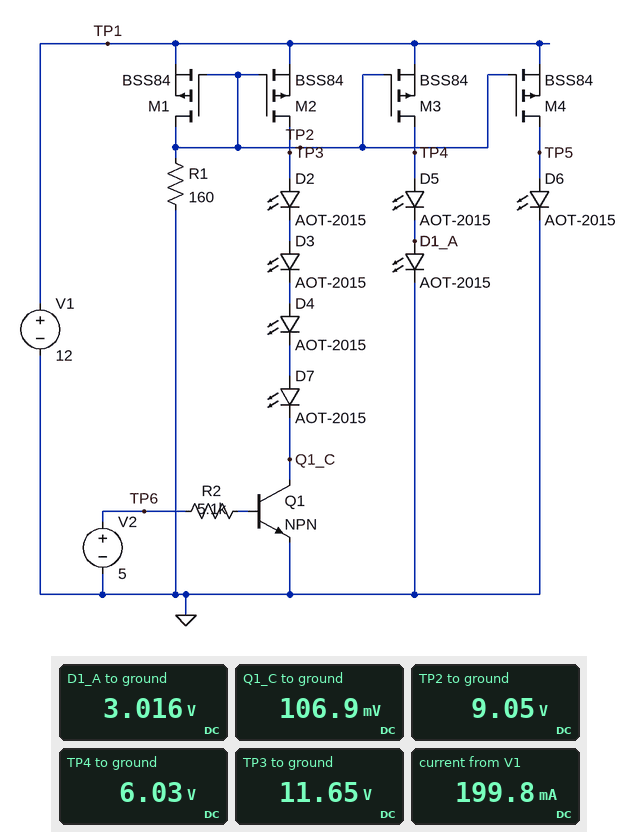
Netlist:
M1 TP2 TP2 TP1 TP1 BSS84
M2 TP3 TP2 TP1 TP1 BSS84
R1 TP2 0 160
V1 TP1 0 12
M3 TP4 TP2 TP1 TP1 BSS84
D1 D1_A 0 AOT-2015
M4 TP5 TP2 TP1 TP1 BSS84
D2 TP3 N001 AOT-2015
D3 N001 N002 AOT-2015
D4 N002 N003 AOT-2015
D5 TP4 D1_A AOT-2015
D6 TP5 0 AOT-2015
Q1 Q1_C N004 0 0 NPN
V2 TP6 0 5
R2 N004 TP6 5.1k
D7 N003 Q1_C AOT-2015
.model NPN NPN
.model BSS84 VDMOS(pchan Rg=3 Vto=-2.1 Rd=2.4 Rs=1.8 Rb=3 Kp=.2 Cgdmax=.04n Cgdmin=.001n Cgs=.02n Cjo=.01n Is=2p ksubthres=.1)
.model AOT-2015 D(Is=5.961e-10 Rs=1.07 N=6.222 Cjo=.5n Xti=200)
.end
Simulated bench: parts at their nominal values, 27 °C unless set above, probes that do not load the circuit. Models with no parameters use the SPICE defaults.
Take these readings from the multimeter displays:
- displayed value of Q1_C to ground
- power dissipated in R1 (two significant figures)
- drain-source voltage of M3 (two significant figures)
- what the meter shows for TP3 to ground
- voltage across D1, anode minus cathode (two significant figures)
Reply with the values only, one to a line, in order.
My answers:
106.9 mV
510 mW
-6.0 V
11.65 V
3.0 V
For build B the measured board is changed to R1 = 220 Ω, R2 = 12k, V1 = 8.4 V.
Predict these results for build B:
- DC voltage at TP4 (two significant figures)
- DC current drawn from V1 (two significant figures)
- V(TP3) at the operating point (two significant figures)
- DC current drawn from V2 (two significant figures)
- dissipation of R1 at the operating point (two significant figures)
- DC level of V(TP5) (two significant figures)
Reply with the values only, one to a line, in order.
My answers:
5.7 V
79 mA
8.4 V
350 µA
150 mW
2.9 V
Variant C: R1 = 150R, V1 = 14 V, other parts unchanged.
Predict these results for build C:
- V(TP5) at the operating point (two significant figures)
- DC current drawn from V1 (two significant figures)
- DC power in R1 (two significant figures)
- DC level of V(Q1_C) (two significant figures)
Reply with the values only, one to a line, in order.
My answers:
3.1 V
290 mA
790 mW
180 mV
